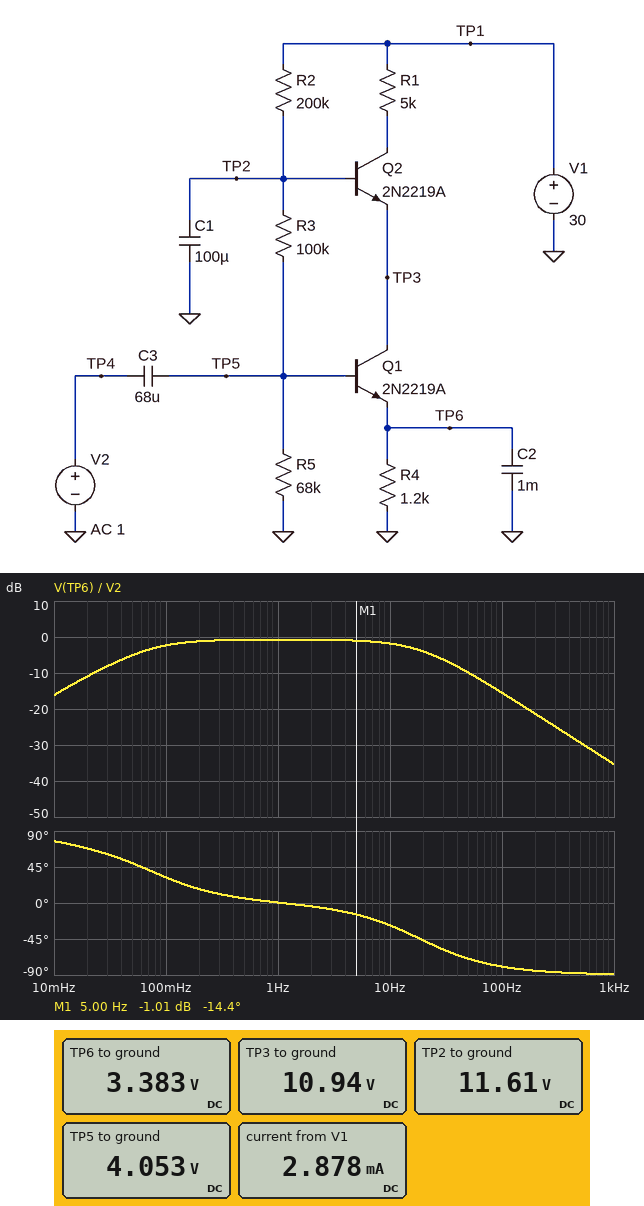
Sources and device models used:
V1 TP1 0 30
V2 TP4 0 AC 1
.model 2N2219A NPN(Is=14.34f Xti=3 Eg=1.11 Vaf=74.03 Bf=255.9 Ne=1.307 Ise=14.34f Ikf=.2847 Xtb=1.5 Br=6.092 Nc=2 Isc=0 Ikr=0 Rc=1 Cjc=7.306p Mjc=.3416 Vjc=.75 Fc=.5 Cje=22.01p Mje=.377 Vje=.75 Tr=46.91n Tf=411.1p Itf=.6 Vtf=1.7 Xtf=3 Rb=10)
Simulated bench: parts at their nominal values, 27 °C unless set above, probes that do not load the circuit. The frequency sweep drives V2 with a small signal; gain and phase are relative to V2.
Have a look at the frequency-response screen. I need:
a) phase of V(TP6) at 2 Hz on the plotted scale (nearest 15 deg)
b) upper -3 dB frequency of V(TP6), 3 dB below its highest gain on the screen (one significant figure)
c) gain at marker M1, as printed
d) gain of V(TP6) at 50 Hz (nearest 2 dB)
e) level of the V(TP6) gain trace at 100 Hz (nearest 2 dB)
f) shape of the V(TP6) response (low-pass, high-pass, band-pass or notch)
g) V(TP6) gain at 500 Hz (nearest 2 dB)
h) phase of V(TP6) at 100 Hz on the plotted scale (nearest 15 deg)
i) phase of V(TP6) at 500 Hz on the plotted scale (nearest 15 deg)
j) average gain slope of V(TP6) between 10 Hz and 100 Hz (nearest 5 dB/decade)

0 deg
20 Hz
-1.01 dB
-10 dB
-16 dB
band-pass
-30 dB
-75 deg
-90 deg
-15 dB/decade
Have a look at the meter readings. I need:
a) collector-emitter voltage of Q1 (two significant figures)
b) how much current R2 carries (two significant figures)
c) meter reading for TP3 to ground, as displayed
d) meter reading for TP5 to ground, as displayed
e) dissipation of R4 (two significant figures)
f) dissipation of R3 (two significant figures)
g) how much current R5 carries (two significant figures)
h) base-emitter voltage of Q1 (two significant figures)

7.6 V
92 µA
10.94 V
4.053 V
9.5 mW
570 µW
60 µA
670 mV
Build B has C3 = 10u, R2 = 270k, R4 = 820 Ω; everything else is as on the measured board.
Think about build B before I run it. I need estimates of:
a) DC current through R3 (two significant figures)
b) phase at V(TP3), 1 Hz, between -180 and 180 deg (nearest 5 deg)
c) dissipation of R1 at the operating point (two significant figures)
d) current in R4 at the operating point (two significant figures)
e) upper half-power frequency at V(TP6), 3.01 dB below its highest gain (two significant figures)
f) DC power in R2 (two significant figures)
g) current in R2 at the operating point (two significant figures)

61 µA
-120 deg
40 mW
2.9 mA
28 Hz
1.6 mW
77 µA
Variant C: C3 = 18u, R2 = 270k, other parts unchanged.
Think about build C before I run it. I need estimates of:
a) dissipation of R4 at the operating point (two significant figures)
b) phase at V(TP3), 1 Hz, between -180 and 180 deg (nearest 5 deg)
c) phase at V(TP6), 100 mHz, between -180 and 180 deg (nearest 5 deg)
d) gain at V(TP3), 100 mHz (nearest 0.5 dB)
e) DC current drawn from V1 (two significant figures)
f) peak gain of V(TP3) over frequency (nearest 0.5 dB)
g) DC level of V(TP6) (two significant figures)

6.1 mW
-120 deg
60 deg
-28.5 dB
2.3 mA
1.0 dB
2.7 V
